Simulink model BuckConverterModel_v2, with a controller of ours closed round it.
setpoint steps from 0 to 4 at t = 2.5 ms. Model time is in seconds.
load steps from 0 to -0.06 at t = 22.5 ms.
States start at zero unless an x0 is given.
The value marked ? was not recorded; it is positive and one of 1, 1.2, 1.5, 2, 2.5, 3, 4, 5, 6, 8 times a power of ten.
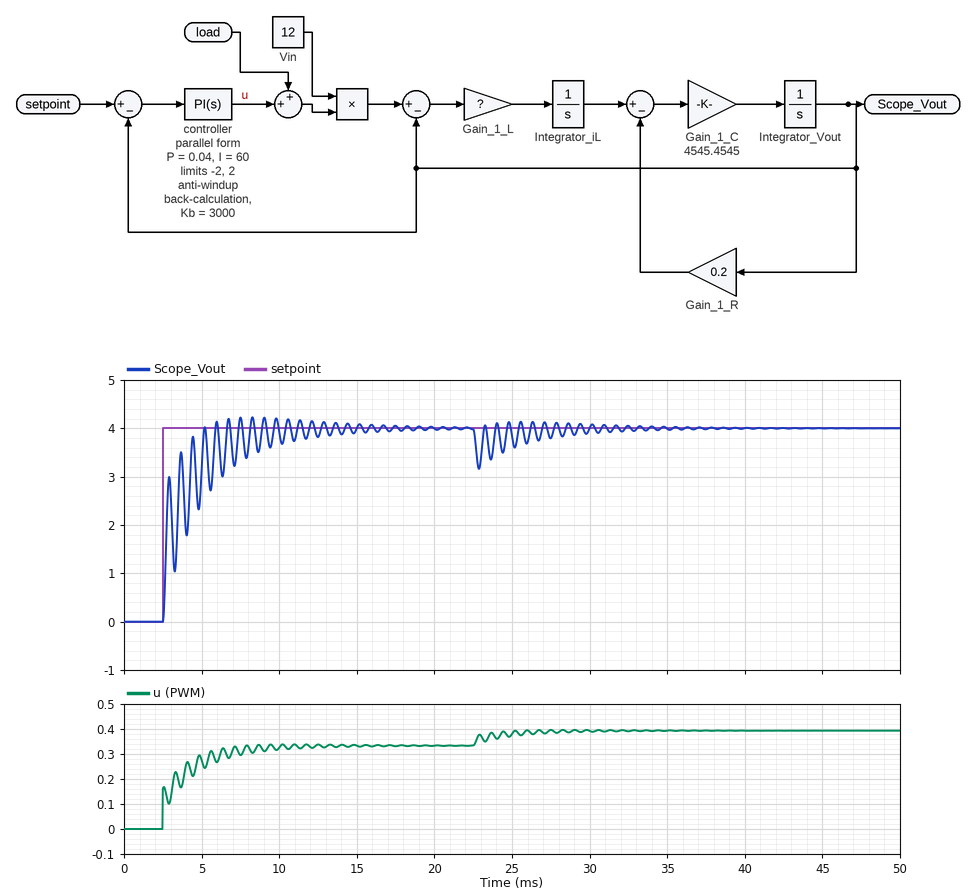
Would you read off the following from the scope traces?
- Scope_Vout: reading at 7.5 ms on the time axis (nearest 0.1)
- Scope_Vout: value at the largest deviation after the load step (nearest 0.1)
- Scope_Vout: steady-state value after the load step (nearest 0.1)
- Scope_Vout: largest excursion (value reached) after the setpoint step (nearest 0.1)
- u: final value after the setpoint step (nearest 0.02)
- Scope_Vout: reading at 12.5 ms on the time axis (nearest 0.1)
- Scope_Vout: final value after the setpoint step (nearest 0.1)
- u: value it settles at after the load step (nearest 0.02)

4.2
3.2
4.0
4.2
0.34
3.8
4.0
0.40
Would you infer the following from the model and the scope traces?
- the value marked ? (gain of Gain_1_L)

10000
